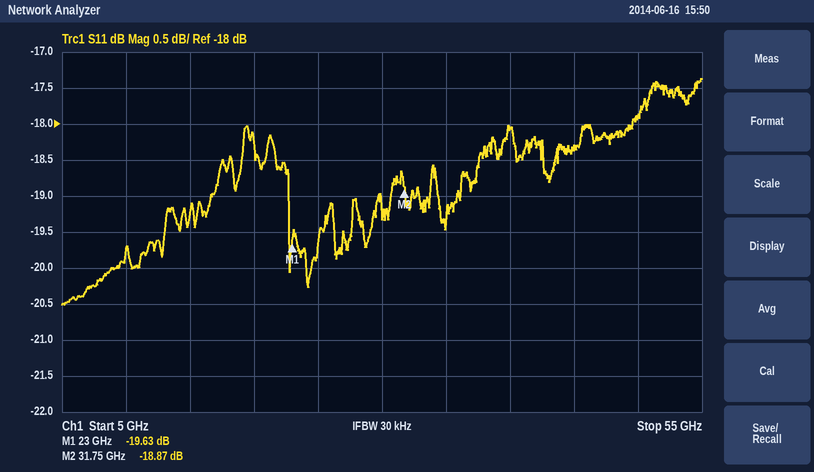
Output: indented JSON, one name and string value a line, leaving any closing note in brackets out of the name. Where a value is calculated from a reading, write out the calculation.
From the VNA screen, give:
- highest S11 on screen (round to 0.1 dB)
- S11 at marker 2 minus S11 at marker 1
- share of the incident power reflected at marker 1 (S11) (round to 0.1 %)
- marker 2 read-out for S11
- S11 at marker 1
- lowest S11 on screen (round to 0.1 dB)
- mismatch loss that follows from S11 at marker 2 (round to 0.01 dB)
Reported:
{
  "highest S11 on screen": "-17.4 dB",
  "S11 at marker 2 minus S11 at marker 1": "-18.87 − (-19.63) = 0.76 dB",
  "share of the incident power reflected at marker 1 (S11)": "10^(-19.63/10) ≈ 1.1 %",
  "marker 2 read-out for S11": "-18.87 dB",
  "S11 at marker 1": "-19.63 dB",
  "lowest S11 on screen": "-20.5 dB",
  "mismatch loss that follows from S11 at marker 2": "−10 log10(1 − 10^(-18.87/10)) ≈ 0.06 dB"
}
